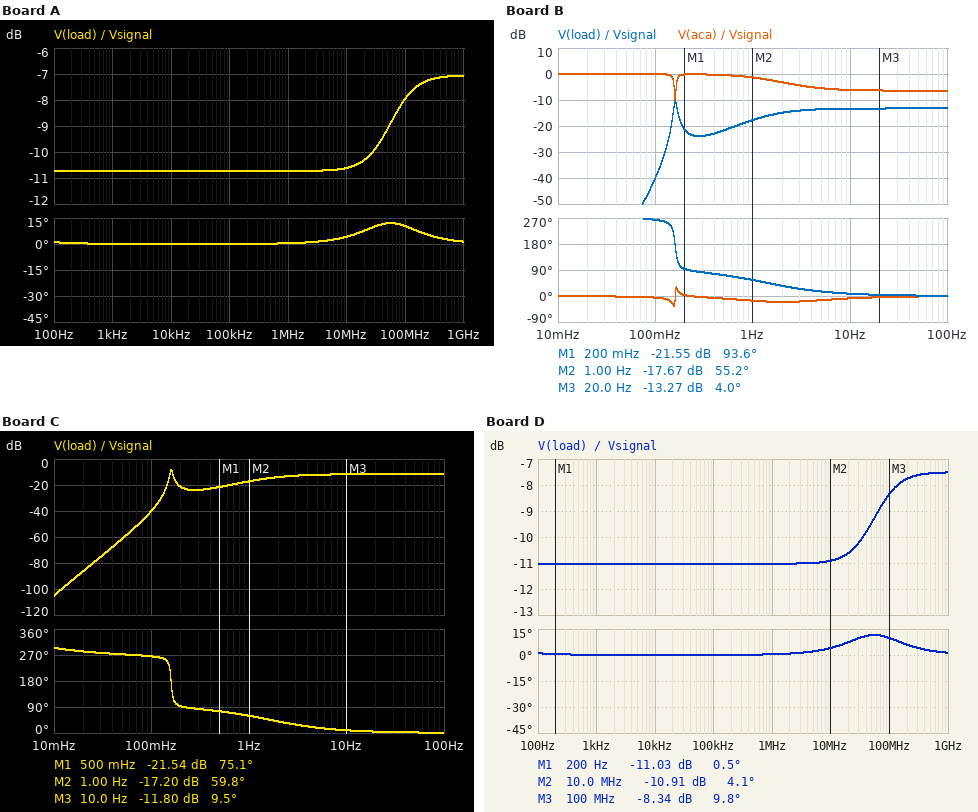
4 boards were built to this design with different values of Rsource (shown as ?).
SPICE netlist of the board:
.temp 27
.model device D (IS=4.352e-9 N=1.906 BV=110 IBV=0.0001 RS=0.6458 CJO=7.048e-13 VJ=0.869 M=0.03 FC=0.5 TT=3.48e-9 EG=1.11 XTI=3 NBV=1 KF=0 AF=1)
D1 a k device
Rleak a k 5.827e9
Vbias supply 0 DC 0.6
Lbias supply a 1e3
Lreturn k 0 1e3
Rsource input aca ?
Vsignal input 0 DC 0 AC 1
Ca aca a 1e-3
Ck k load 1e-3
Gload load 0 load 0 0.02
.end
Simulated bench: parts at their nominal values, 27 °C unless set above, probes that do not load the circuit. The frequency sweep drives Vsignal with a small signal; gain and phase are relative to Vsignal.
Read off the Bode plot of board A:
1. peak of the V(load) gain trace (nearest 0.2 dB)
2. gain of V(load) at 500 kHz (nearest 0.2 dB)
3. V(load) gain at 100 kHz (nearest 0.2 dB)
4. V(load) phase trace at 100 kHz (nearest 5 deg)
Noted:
-7.0 dB
-10.8 dB
-10.8 dB
0 deg
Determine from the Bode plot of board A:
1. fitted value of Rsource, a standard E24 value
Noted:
62 Ω
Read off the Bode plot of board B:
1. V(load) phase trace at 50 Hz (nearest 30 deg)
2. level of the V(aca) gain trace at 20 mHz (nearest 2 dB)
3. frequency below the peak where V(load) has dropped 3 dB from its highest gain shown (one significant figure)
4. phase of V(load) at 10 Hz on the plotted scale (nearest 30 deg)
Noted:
0 deg
0 dB
200 mHz
0 deg
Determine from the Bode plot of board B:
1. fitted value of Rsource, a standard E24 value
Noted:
120 Ω
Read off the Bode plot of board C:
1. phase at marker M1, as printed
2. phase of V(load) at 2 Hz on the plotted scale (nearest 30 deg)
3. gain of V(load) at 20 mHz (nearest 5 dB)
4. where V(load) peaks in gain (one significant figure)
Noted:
75.1 deg
30 deg
-85 dB
200 mHz
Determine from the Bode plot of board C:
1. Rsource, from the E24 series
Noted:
82 Ω
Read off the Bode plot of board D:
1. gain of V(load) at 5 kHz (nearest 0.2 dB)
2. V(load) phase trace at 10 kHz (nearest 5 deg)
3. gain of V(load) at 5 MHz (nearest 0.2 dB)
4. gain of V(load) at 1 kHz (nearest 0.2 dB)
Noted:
-11.0 dB
0 deg
-11.0 dB
-11.0 dB
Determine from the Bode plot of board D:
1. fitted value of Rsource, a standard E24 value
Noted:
68 Ω
